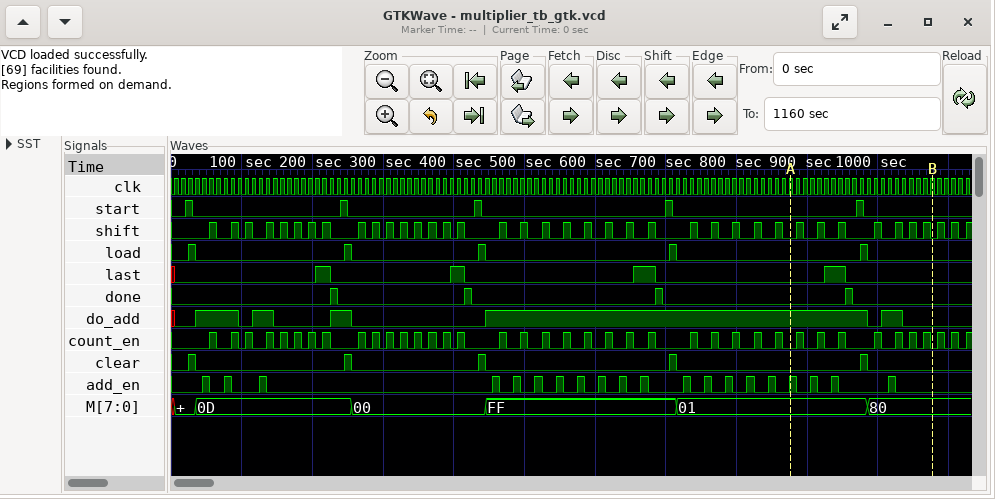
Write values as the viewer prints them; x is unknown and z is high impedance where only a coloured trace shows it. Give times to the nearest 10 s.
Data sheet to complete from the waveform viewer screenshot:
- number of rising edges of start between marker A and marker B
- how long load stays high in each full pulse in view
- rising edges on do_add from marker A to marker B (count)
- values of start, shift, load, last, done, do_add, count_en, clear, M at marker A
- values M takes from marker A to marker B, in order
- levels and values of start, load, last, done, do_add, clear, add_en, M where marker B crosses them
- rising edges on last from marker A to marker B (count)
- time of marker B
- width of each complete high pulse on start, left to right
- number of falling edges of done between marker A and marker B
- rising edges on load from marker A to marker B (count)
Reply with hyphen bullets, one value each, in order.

- 1
- 10 s, 10 s, 10 s, 10 s, 10 s
- 1
- start=0, shift=0, load=0, last=0, done=0, do_add=1, count_en=0, clear=0, M=01
- 01, 80
- start=0, load=0, last=0, done=0, do_add=0, clear=0, add_en=0, M=80
- 1
- 1080 s
- 10 s, 10 s, 10 s, 10 s, 10 s
- 1
- 1
